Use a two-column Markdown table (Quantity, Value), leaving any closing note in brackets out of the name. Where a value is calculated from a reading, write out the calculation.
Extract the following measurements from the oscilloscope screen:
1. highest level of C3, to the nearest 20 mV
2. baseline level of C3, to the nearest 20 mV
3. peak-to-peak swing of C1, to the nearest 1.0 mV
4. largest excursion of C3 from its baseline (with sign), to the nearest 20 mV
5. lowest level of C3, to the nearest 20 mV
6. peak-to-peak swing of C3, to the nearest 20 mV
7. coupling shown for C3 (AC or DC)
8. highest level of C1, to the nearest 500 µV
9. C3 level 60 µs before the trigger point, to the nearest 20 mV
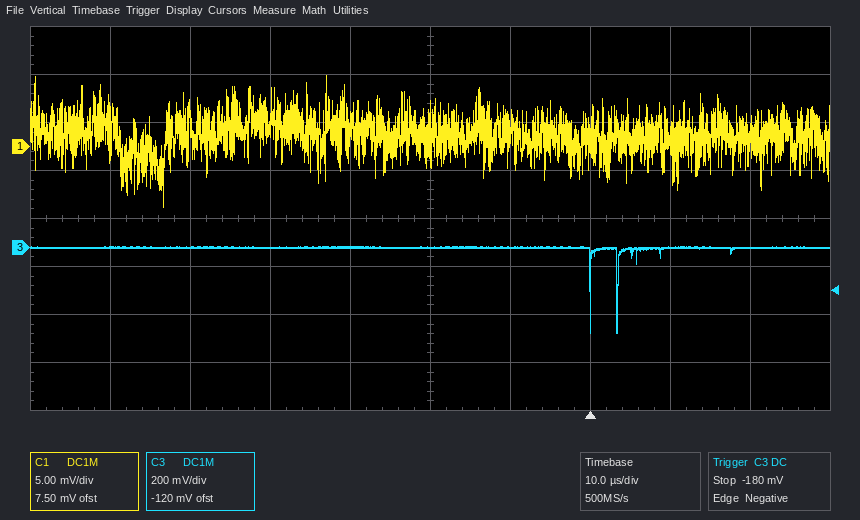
| Quantity | Value |
|---|---|
| highest level of C3, to the nearest 20 mV | 0 mV |
| baseline level of C3, to the nearest 20 mV | 0 mV |
| peak-to-peak swing of C1, to the nearest 1.0 mV | 14.0 mV |
| largest excursion of C3 from its baseline (with sign), to the nearest 20 mV | -360 mV − (0 mV) = -360 mV |
| lowest level of C3, to the nearest 20 mV | -360 mV |
| peak-to-peak swing of C3, to the nearest 20 mV | 0 mV − (-360 mV) = 360 mV |
| coupling shown for C3 | DC |
| highest level of C1, to the nearest 500 µV | 7.5 mV |
| C3 level 60 µs before the trigger point, to the nearest 20 mV | 0 mV |
